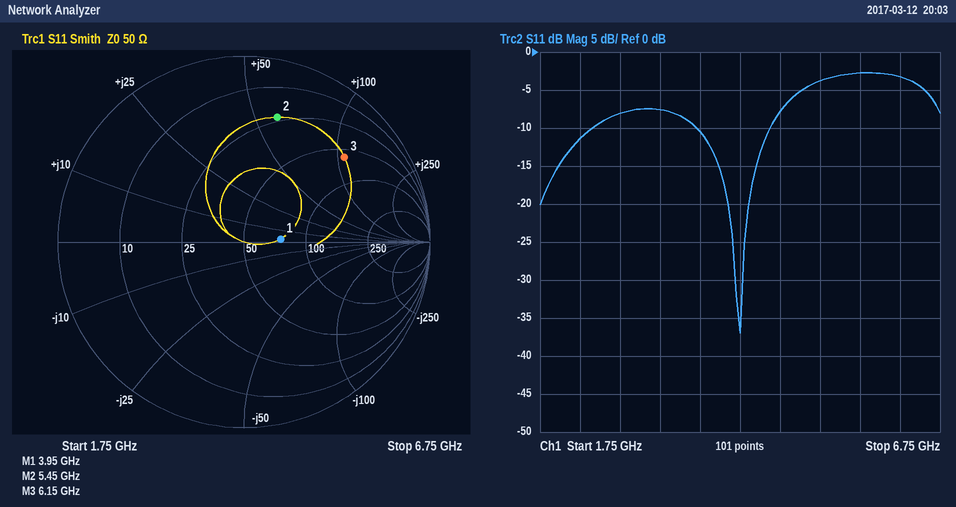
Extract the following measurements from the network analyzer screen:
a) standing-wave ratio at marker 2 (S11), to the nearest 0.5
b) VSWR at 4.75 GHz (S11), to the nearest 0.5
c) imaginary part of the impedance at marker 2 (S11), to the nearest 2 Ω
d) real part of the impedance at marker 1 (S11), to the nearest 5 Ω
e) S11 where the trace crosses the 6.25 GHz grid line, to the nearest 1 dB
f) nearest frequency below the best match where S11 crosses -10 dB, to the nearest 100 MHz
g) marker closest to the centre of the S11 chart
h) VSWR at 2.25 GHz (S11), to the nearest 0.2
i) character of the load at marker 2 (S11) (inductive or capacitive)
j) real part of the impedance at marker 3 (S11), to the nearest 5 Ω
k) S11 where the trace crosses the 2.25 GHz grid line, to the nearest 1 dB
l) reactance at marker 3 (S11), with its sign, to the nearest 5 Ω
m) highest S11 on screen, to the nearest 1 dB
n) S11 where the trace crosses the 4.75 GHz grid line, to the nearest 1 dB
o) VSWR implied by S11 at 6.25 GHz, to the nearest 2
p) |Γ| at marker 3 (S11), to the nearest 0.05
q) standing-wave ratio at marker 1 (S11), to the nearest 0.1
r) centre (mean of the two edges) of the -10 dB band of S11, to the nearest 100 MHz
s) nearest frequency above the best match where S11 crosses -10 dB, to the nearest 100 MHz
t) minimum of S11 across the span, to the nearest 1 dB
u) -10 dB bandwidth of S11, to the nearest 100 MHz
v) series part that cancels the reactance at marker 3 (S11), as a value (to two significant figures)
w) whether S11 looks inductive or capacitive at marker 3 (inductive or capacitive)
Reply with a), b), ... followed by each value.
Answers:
a) 5.5
b) 2.5
c) +60 Ω
d) 75 Ω
e) -3 dB
f) 3.7 GHz
g) marker 1
h) 1.8
i) inductive
j) 60 Ω
k) -11 dB
l) +110 Ω
m) -3 dB
n) -8 dB
o) 6
p) 0.70
q) 1.5
r) 4.2 GHz
s) 4.6 GHz
t) -37 dB
u) 900 MHz
v) 240 fF
w) inductive
